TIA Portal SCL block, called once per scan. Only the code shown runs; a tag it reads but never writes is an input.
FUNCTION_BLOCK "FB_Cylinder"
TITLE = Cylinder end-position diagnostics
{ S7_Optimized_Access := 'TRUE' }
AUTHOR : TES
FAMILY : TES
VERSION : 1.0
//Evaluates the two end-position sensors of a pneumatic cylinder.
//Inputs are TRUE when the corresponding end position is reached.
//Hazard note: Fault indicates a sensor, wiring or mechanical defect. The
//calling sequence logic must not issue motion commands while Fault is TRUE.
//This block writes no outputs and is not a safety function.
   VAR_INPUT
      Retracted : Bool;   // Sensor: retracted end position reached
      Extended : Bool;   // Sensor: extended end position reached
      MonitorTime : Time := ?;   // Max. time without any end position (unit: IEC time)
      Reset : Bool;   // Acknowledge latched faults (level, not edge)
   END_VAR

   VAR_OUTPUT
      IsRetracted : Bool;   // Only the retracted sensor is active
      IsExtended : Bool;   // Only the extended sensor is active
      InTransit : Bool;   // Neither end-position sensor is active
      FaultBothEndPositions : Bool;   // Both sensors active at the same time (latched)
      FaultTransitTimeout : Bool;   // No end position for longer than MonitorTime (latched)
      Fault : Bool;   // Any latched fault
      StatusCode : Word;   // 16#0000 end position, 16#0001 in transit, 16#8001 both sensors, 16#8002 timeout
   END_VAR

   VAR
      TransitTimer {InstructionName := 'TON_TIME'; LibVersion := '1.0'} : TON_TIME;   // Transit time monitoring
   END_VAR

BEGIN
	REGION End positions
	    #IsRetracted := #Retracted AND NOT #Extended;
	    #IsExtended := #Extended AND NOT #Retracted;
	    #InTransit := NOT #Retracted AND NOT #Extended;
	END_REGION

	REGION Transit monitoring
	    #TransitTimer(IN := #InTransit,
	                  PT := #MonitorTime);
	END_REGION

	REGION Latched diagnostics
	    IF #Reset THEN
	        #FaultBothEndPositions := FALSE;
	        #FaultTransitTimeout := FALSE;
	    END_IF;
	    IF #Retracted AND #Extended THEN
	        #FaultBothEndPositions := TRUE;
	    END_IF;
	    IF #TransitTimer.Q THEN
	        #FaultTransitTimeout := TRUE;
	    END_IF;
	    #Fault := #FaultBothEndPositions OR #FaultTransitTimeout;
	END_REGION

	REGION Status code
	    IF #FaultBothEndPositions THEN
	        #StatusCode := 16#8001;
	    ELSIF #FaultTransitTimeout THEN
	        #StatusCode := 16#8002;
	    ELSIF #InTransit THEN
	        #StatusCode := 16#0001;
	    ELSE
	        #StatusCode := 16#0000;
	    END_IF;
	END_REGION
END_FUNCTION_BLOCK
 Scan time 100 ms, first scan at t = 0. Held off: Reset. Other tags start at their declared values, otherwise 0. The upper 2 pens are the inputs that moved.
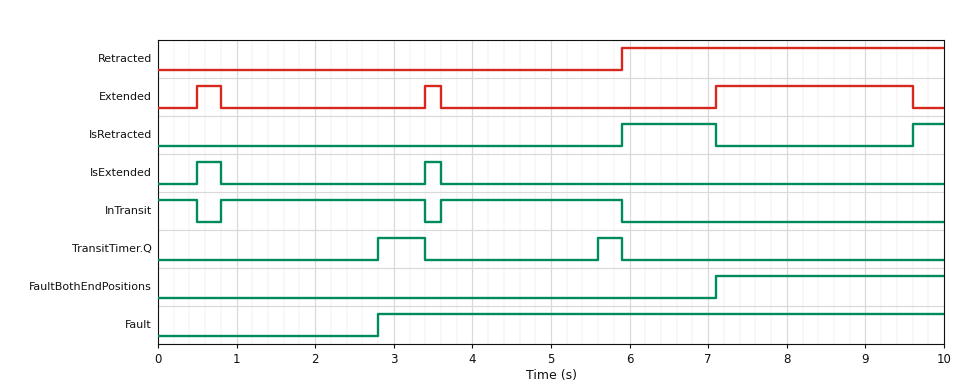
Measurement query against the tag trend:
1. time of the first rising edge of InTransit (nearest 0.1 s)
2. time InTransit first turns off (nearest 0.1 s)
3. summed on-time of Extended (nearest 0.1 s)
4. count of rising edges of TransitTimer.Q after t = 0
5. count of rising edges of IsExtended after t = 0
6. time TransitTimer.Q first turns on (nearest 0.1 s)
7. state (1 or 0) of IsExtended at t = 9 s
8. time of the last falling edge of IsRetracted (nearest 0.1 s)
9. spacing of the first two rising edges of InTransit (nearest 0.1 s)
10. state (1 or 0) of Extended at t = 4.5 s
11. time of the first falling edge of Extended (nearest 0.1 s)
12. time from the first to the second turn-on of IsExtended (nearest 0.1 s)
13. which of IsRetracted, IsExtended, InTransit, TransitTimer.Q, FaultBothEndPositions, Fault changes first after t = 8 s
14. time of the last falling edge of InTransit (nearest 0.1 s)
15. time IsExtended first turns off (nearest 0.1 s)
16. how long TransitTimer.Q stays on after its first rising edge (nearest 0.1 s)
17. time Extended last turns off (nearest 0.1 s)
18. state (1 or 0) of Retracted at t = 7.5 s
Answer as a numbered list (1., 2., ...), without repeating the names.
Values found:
1. 0.8 s
2. 0.5 s
3. 3.0 s
4. 2
5. 2
6. 2.8 s
7. 0
8. 7.1 s
9. 2.8 s
10. 0
11. 0.8 s
12. 2.9 s
13. IsRetracted
14. 5.9 s
15. 0.8 s
16. 0.6 s
17. 9.6 s
18. 1
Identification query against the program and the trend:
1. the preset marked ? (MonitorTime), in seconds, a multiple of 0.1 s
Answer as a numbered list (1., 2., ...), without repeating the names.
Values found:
1. 2.0 s
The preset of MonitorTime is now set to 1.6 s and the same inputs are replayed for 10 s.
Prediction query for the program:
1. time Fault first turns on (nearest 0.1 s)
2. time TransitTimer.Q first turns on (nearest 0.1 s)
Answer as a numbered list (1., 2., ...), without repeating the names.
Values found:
1. 2.4 s
2. 2.4 s
